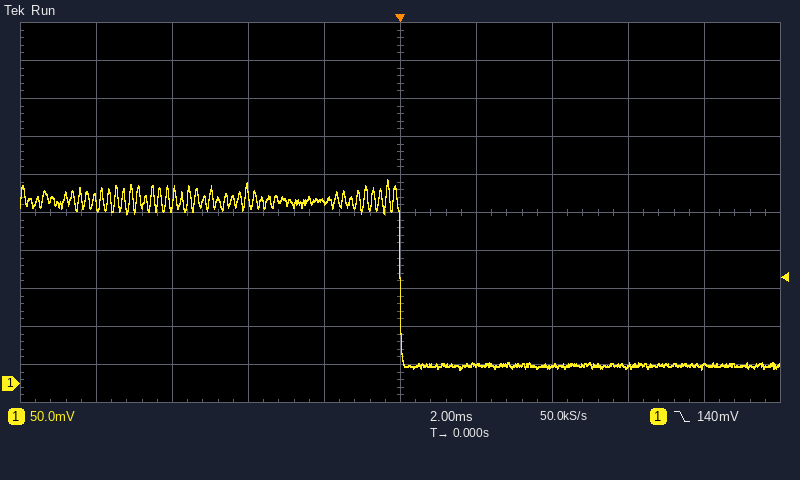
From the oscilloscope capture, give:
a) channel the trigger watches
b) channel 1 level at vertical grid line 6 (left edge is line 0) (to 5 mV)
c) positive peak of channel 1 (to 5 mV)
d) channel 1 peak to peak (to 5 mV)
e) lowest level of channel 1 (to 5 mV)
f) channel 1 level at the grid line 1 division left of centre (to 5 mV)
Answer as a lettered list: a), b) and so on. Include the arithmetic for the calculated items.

a) channel 1
b) 25 mV
c) 270 mV
d) 270 mV − (20 mV) = 250 mV
e) 20 mV
f) 240 mV
